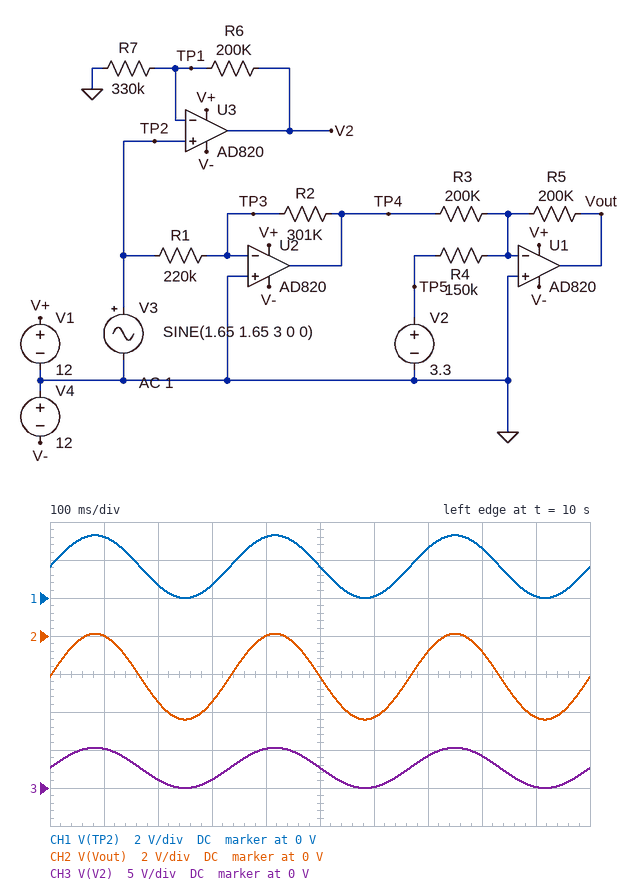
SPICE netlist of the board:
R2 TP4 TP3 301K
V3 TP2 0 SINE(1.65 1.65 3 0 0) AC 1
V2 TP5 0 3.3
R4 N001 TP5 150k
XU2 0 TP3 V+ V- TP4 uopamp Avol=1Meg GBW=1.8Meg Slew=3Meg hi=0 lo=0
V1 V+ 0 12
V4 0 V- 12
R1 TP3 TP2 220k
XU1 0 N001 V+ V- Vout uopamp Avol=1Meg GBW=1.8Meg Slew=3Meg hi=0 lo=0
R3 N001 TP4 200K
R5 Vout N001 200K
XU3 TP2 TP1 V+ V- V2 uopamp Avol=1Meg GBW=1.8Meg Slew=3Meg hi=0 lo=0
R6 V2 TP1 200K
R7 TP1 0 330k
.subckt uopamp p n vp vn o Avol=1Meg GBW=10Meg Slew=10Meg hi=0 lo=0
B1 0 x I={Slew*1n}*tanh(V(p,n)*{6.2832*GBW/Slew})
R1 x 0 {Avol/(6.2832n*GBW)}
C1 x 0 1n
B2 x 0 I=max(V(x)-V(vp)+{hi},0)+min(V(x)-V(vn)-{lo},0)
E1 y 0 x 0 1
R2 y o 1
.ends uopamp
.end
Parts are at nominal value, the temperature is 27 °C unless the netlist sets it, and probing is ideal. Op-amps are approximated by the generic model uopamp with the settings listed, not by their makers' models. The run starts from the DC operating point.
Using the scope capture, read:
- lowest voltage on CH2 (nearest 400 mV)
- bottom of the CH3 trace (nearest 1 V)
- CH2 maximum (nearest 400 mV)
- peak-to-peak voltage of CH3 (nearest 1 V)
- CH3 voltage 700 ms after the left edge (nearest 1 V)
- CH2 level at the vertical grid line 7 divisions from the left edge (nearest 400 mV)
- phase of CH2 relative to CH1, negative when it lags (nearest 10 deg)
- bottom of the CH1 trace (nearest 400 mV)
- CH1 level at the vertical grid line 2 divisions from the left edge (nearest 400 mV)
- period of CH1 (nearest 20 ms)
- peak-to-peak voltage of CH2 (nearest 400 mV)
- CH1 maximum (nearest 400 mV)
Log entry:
-4.4 V
0 V
0 V
5 V
4 V
-800 mV
0 deg
0 V
800 mV
340 ms
4.4 V
3.2 V
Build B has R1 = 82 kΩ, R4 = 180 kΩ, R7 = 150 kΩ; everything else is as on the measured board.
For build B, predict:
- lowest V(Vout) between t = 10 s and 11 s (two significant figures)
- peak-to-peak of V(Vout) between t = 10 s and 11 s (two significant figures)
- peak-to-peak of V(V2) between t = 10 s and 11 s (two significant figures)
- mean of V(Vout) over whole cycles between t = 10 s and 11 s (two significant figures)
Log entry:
-3.7 V
12 V
7.7 V
2.4 V
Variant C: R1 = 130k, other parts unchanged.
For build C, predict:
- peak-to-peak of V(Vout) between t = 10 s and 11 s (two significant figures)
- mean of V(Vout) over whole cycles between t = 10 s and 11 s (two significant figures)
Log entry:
7.6 V
-580 mV
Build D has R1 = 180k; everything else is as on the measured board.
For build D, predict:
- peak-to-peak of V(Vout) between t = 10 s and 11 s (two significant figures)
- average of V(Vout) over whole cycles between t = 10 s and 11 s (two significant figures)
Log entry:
5.5 V
-1.6 V
